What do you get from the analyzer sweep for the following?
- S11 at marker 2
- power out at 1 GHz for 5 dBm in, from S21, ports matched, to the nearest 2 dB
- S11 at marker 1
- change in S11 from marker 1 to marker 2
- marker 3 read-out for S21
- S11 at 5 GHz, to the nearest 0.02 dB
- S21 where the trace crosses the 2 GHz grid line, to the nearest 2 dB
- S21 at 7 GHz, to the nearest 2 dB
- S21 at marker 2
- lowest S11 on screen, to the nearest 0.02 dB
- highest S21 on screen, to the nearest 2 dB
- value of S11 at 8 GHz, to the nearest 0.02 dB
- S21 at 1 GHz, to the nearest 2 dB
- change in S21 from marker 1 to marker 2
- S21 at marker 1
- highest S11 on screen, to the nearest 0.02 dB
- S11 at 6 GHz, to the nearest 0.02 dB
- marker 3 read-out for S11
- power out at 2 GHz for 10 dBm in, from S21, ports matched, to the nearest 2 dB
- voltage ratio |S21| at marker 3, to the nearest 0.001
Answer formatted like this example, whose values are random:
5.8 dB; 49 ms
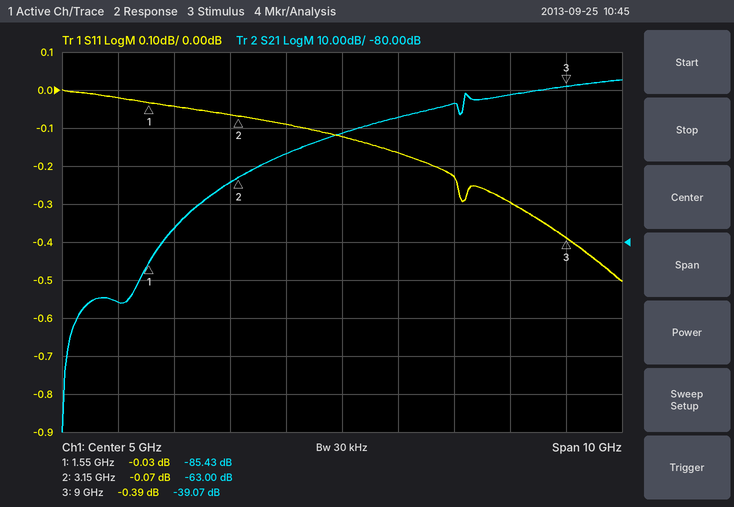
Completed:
-0.07 dB; -90 dBm; -0.03 dB; -0.04 dB; -39.07 dB; -0.12 dB; -76 dB; -44 dB; -63.00 dB; -0.50 dB; -38 dB; -0.30 dB; -96 dB; 22.43 dB; -85.43 dB; 0.00 dB; -0.16 dB; -0.39 dB; -66 dBm; 0.011
